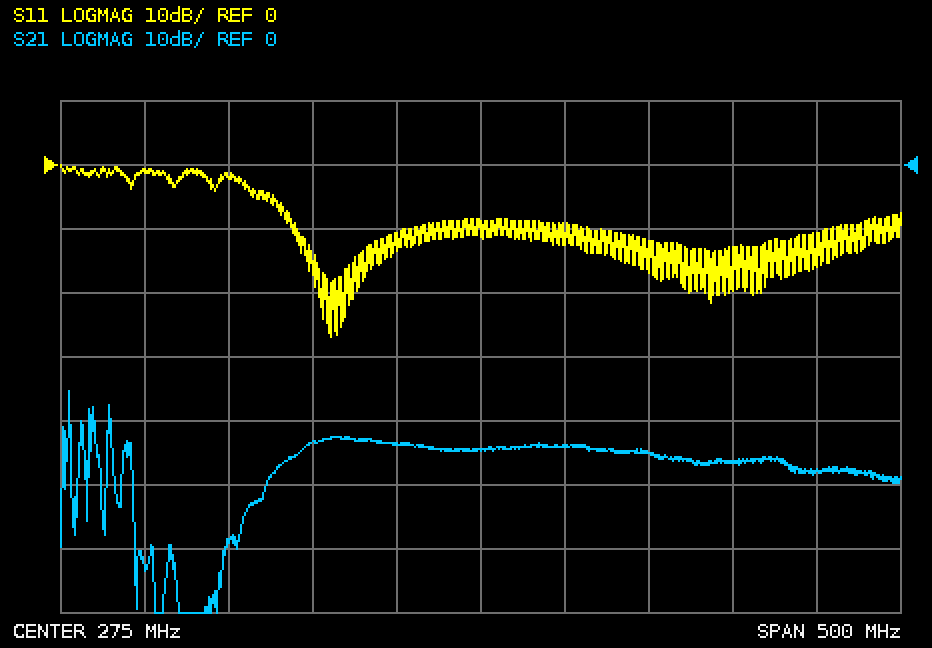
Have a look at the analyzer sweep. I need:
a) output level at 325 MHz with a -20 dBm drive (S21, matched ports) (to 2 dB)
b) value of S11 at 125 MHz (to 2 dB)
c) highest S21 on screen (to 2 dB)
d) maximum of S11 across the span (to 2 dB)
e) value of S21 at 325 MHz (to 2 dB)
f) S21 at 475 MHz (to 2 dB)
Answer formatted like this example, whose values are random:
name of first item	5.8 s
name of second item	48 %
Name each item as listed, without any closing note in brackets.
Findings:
output level at 325 MHz with a -20 dBm drive (S21, matched ports)	-64 dBm
value of S11 at 125 MHz	-2 dB
highest S21 on screen	-36 dB
maximum of S11 across the span	0 dB
value of S21 at 325 MHz	-44 dB
S21 at 475 MHz	-48 dB
